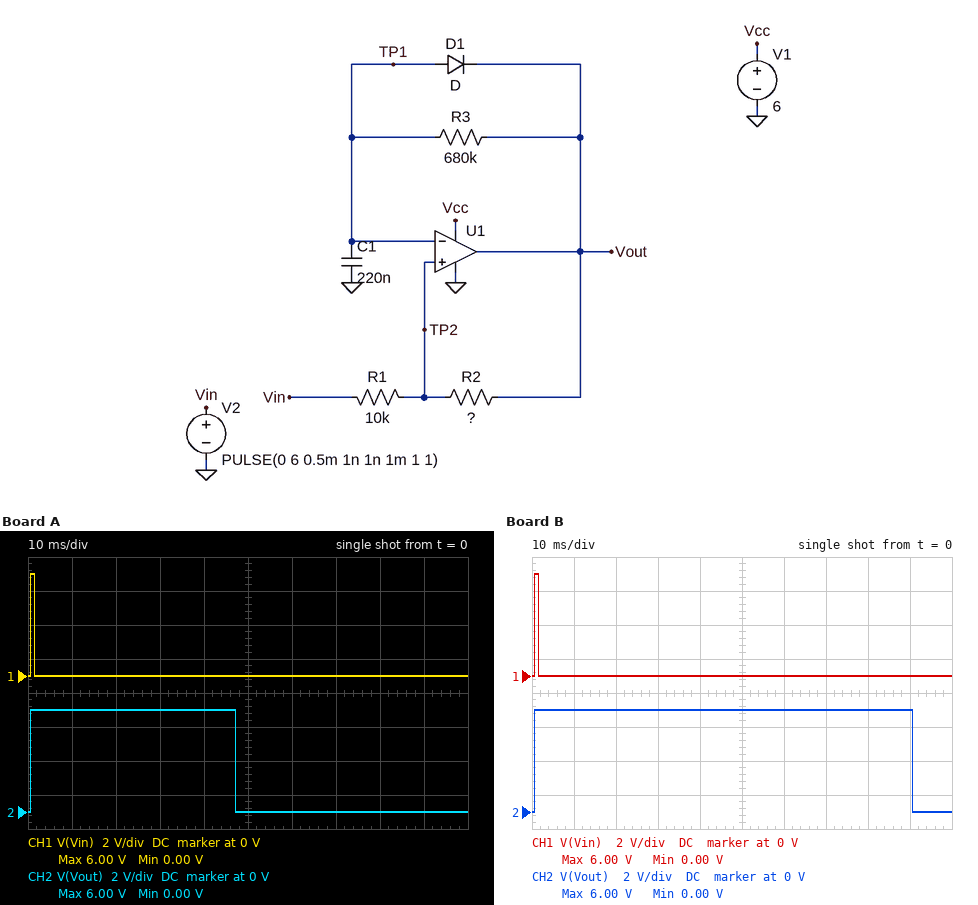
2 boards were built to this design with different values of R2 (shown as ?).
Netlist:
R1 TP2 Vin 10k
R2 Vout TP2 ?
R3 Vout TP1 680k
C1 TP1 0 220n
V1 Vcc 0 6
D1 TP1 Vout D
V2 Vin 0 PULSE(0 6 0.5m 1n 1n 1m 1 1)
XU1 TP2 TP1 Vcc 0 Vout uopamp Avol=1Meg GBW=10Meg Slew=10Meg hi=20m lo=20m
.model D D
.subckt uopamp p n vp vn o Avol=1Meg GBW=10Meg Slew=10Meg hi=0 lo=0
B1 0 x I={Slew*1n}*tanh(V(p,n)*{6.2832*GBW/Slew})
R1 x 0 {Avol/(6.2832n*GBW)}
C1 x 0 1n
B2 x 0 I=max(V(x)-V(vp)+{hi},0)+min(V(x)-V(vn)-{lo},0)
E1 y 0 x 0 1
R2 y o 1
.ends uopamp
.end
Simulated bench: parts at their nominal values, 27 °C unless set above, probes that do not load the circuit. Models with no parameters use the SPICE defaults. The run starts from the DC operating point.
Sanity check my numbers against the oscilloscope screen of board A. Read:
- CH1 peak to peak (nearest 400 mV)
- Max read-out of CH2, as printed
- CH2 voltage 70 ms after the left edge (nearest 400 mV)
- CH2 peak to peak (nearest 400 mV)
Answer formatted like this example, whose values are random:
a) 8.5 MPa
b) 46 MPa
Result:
a) 6.0 V
b) 6.00 V
c) 0 V
d) 6.0 V
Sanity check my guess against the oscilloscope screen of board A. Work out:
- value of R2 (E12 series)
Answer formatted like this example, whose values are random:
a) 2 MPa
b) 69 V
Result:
a) 27 kΩ
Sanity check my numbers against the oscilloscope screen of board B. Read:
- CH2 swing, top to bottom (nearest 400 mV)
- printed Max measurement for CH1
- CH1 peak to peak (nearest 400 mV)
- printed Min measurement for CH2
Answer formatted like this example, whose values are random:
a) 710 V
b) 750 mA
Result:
a) 6.0 V
b) 6.00 V
c) 6.0 V
d) 0.00 V
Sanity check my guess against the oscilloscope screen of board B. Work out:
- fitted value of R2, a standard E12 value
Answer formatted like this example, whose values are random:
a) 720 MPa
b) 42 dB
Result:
a) 12 kΩ
